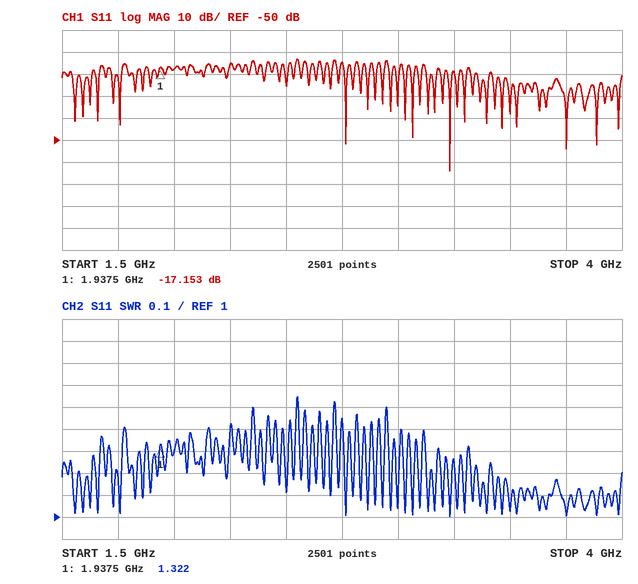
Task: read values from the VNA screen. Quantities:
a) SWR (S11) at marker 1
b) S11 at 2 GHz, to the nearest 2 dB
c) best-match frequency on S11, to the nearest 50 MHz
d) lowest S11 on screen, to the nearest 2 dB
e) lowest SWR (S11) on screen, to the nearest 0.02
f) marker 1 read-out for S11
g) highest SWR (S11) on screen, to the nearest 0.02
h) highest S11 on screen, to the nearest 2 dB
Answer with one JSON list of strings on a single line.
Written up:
["1.322", "-18 dB", "3.25 GHz", "-64 dB", "1.00", "-17.153 dB", "1.54", "-14 dB"]
